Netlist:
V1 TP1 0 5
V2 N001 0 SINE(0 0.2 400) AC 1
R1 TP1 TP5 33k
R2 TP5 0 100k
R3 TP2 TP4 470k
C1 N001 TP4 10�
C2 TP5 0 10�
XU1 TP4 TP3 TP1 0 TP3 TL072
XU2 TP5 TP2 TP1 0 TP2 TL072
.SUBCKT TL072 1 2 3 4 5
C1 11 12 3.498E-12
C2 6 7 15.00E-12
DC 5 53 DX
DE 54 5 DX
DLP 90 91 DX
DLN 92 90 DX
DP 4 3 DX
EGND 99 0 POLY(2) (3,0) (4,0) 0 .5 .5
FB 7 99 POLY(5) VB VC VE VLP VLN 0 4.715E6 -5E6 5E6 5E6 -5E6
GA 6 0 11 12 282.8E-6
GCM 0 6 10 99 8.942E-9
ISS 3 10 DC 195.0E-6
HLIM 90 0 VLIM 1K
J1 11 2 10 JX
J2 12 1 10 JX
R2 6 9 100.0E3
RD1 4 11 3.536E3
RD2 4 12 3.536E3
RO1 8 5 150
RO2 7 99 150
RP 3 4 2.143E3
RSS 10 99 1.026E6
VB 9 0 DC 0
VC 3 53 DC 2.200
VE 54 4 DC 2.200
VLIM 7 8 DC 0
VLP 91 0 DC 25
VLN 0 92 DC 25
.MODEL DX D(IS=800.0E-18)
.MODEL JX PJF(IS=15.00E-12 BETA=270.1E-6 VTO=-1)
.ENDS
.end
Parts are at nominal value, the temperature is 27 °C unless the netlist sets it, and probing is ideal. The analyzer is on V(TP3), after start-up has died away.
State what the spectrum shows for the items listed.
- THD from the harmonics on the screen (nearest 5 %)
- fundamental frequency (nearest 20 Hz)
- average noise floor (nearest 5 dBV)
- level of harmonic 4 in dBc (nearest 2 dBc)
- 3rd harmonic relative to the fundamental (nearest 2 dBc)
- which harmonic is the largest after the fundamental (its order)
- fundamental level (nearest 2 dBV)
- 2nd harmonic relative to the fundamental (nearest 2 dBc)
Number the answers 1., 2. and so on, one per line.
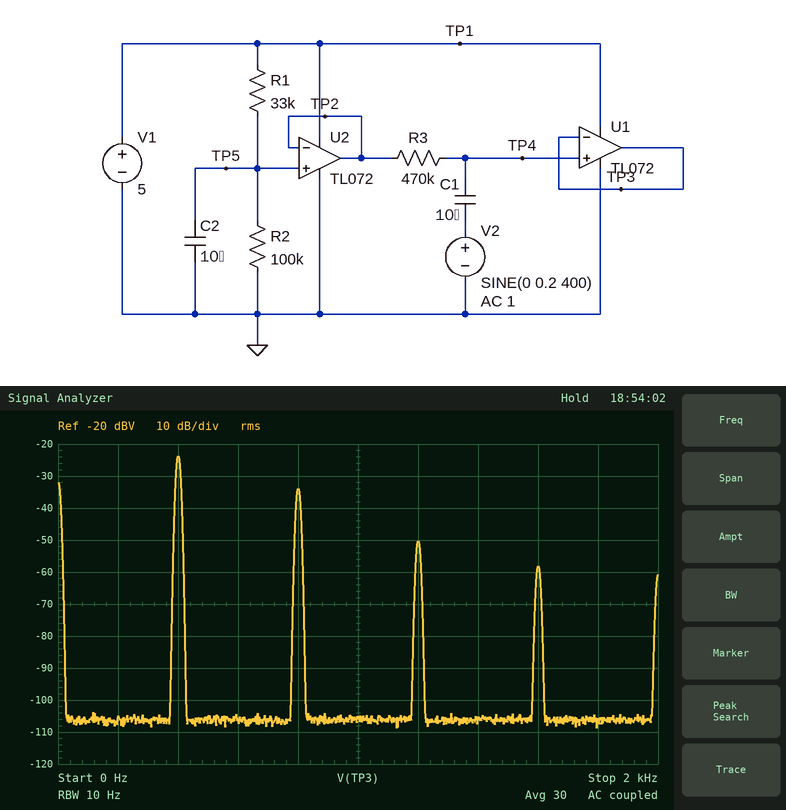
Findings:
1. 30 %
2. 400 Hz
3. -105 dBV
4. -34 dBc
5. -26 dBc
6. 2
7. -24 dBV
8. -10 dBc
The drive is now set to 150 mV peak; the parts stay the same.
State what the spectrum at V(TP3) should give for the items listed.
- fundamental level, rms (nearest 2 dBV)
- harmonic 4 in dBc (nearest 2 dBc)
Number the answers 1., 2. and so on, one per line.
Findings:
1. -26 dBV
2. -44 dBc
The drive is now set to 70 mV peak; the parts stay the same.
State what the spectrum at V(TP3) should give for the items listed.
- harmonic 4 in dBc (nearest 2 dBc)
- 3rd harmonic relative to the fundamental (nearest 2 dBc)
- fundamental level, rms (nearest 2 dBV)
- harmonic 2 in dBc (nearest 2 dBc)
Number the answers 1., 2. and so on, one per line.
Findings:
1. -58 dBc
2. -34 dBc
3. -34 dBV
4. -16 dBc
